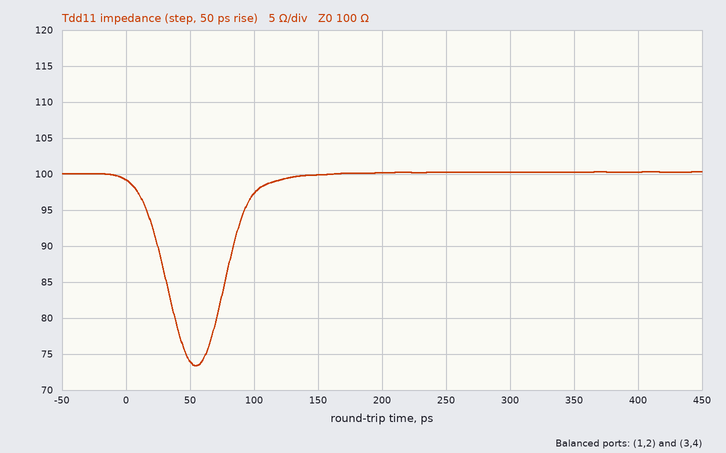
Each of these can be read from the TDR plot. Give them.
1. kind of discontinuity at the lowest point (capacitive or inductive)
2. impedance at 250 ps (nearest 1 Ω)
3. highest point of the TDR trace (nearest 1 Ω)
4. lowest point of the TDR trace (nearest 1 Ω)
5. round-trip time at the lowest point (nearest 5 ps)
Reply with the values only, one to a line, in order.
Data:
capacitive
100 Ω
100 Ω
73 Ω
55 ps
